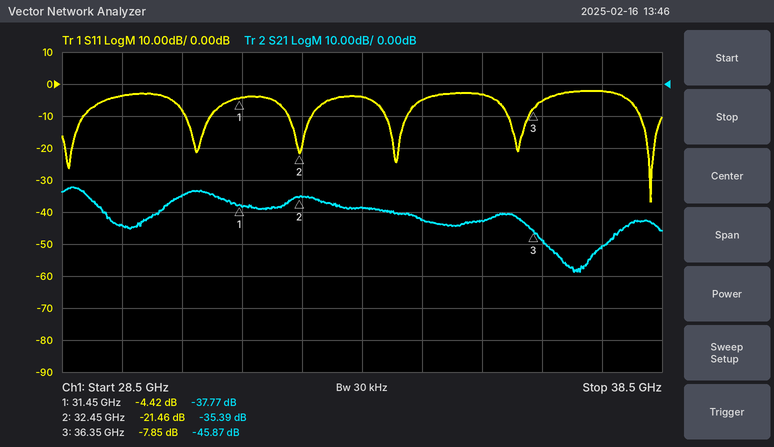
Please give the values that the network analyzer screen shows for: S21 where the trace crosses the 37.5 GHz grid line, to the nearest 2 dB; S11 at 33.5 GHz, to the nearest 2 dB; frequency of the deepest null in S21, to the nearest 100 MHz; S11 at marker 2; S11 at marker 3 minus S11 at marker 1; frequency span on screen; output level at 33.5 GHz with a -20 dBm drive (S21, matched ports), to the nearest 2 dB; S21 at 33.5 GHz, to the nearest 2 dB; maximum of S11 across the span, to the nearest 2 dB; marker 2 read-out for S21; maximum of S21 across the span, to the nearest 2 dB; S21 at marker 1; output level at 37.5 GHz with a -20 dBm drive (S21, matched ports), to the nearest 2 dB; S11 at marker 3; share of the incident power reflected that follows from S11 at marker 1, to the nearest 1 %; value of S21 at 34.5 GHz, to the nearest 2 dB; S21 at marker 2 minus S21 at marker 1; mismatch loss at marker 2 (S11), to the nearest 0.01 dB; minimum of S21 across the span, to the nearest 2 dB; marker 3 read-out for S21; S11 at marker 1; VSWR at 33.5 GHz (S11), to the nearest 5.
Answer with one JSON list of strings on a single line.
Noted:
["-50 dB", "-4 dB", "37.0 GHz", "-21.46 dB", "-3.43 dB", "10 GHz", "-58 dBm", "-38 dB", "-2 dB", "-35.39 dB", "-32 dB", "-37.77 dB", "-70 dBm", "-7.85 dB", "36 %", "-42 dB", "2.38 dB", "0.03 dB", "-58 dB", "-45.87 dB", "-4.42 dB", "5"]
